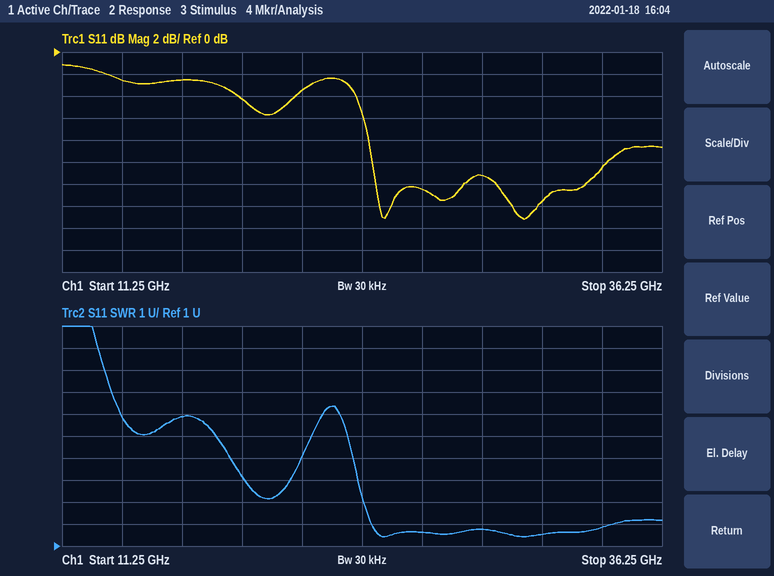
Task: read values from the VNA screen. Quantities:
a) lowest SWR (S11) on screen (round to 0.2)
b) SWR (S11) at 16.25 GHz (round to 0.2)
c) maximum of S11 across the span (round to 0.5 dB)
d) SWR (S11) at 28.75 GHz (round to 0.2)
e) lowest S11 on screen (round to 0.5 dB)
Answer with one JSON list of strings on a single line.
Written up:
["1.4", "6.8", "-1.0 dB", "1.8", "-15.0 dB"]
